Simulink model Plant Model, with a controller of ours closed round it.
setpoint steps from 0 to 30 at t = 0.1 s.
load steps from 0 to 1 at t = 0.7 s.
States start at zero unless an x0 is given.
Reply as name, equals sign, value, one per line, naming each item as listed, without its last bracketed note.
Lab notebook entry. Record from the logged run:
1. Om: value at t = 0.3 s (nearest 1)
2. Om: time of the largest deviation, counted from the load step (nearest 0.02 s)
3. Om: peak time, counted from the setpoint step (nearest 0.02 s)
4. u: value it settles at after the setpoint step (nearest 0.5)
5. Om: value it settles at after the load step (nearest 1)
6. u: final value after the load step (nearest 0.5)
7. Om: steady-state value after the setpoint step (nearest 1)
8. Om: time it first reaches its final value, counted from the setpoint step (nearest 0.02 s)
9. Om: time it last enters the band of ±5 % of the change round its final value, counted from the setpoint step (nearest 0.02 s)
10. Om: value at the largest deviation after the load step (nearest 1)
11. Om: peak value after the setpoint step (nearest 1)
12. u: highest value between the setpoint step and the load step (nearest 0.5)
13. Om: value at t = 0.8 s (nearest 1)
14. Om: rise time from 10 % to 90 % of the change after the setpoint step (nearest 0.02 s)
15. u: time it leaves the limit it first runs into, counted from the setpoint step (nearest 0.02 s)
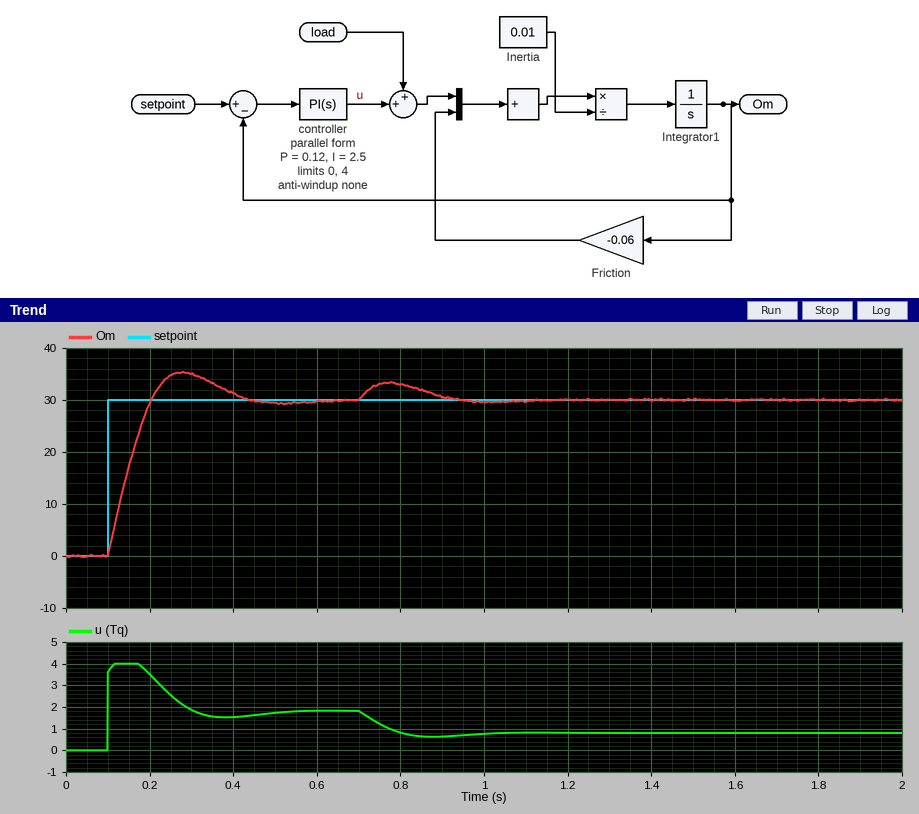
Om: value at t = 0.3 s = 35
Om: time of the largest deviation, counted from the load step = 0.08 s
Om: peak time, counted from the setpoint step = 0.18 s
u: value it settles at after the setpoint step = 2.0
Om: value it settles at after the load step = 30
u: final value after the load step = 1.0
Om: steady-state value after the setpoint step = 30
Om: time it first reaches its final value, counted from the setpoint step = 0.10 s
Om: time it last enters the band of ±5 % of the change round its final value, counted from the setpoint step = 0.30 s
Om: value at the largest deviation after the load step = 33
Om: peak value after the setpoint step = 35
u: highest value between the setpoint step and the load step = 4.0
Om: value at t = 0.8 s = 33
Om: rise time from 10 % to 90 % of the change after the setpoint step = 0.08 s
u: time it leaves the limit it first runs into, counted from the setpoint step = 0.08 s
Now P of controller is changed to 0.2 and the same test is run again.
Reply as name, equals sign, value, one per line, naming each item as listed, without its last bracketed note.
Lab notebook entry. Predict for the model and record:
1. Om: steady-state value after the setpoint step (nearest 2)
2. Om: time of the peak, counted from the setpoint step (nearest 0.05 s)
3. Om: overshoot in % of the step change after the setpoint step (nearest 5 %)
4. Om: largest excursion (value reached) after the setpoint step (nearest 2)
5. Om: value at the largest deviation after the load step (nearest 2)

Om: steady-state value after the setpoint step = 30
Om: time of the peak, counted from the setpoint step = 0.15 s
Om: overshoot in % of the step change after the setpoint step = 15 %
Om: largest excursion (value reached) after the setpoint step = 34
Om: value at the largest deviation after the load step = 32
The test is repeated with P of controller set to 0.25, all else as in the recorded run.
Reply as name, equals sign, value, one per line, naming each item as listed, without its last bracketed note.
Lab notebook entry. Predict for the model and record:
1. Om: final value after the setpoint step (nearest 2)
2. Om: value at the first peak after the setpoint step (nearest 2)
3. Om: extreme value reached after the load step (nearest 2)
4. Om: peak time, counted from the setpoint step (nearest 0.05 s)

Om: final value after the setpoint step = 30
Om: value at the first peak after the setpoint step = 34
Om: extreme value reached after the load step = 32
Om: peak time, counted from the setpoint step = 0.15 s
